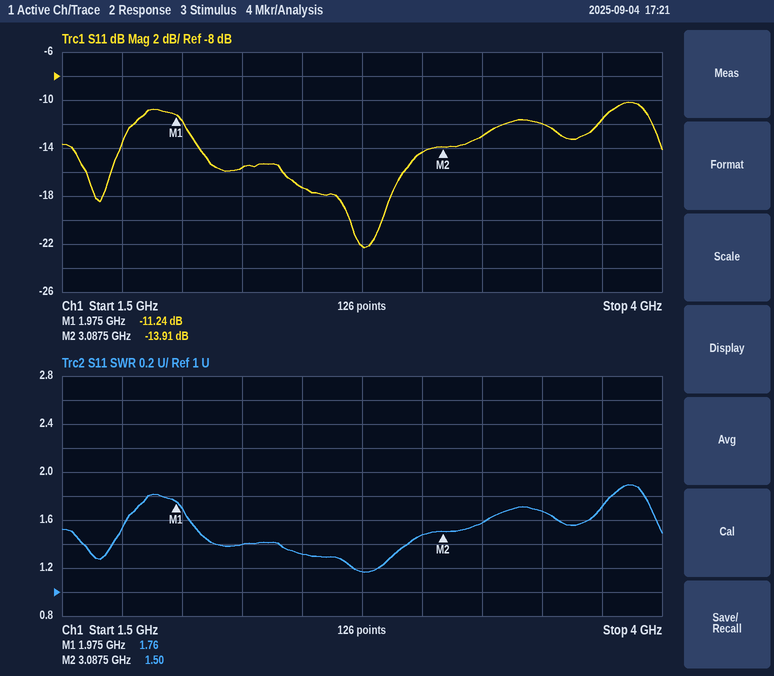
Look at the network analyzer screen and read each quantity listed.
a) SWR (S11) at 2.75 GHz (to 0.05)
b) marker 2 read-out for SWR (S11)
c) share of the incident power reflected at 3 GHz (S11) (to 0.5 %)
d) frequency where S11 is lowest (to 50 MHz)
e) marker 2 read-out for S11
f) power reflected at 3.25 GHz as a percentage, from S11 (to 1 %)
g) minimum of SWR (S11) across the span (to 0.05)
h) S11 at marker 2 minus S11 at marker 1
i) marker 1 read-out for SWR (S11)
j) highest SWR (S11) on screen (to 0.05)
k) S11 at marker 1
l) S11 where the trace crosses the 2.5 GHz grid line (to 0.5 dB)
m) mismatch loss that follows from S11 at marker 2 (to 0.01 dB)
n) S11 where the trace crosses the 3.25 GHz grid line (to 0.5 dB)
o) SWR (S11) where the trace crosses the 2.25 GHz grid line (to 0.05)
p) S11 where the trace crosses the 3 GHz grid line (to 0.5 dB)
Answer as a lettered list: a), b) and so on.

a) 1.15
b) 1.50
c) 3.5 %
d) 2.75 GHz
e) -13.91 dB
f) 5 %
g) 1.15
h) -2.67 dB
i) 1.76
j) 1.90
k) -11.24 dB
l) -17.5 dB
m) 0.18 dB
n) -13.0 dB
o) 1.40
p) -14.5 dB
